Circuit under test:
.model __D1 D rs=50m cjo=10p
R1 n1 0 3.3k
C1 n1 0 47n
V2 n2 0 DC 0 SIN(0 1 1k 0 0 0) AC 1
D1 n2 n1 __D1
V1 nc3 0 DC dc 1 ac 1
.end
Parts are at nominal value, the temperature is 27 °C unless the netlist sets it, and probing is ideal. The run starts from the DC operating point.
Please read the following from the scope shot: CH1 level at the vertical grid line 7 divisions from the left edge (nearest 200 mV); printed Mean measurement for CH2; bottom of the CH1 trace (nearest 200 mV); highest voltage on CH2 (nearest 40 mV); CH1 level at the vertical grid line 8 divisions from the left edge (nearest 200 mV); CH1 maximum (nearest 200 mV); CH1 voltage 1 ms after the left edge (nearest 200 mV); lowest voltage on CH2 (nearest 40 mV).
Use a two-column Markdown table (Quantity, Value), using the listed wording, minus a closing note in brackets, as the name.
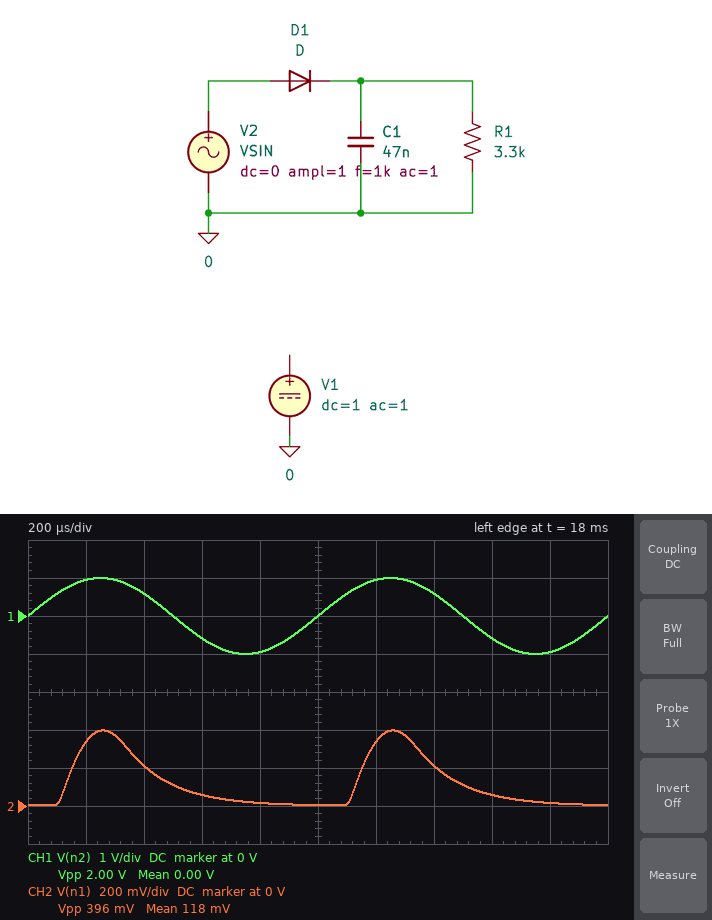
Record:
| Quantity | Value |
|---|---|
| CH1 level at the vertical grid line 7 divisions from the left edge | 600 mV |
| printed Mean measurement for CH2 | 118 mV |
| bottom of the CH1 trace | -1.0 V |
| highest voltage on CH2 | 400 mV |
| CH1 level at the vertical grid line 8 divisions from the left edge | -600 mV |
| CH1 maximum | 1.0 V |
| CH1 voltage 1 ms after the left edge | 0 V |
| lowest voltage on CH2 | 0 V |
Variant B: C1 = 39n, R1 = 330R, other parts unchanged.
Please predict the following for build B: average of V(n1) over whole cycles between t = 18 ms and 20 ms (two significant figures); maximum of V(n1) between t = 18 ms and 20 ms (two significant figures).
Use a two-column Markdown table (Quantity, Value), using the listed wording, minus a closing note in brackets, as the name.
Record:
| Quantity | Value |
|---|---|
| average of V(n1) over whole cycles between t = 18 ms and 20 ms | 66 mV |
| maximum of V(n1) between t = 18 ms and 20 ms | 340 mV |
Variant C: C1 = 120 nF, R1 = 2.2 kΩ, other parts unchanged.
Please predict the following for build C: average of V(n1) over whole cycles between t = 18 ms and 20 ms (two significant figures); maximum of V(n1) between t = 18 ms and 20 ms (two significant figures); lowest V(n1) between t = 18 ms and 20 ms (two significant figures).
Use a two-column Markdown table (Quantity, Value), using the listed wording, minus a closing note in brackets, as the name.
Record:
| Quantity | Value |
|---|---|
| average of V(n1) over whole cycles between t = 18 ms and 20 ms | 150 mV |
| maximum of V(n1) between t = 18 ms and 20 ms | 390 mV |
| lowest V(n1) between t = 18 ms and 20 ms | 19 mV |
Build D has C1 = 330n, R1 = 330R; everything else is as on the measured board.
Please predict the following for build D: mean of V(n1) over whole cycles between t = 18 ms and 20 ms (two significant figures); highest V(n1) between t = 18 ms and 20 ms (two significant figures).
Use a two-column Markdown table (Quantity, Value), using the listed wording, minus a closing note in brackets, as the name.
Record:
| Quantity | Value |
|---|---|
| mean of V(n1) over whole cycles between t = 18 ms and 20 ms | 85 mV |
| highest V(n1) between t = 18 ms and 20 ms | 340 mV |
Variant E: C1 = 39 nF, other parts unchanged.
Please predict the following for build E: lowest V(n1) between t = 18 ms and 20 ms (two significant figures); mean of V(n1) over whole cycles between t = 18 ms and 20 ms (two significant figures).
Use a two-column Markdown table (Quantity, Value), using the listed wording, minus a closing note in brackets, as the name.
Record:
| Quantity | Value |
|---|---|
| lowest V(n1) between t = 18 ms and 20 ms | 1.2 mV |
| mean of V(n1) over whole cycles between t = 18 ms and 20 ms | 110 mV |
